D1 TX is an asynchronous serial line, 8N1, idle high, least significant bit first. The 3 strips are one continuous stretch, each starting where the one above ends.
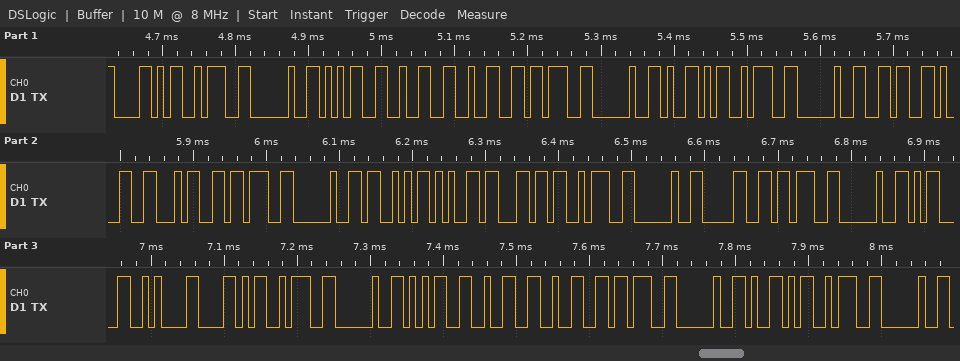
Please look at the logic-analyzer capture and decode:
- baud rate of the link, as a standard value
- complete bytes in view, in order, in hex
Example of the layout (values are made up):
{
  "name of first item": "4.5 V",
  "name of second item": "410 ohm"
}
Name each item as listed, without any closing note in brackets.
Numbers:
{
  "baud rate of the link, as a standard value": "115200 baud",
  "complete bytes in view, in order, in hex": "58 3A 20 35 32 32 3B 20 59 3A 20 36 31 34 3B 20 53 65 6C 3A 20 30 3B 20 0D 0A 58 3A 20 35 32 32 3B 20 59 3A 20"
}
